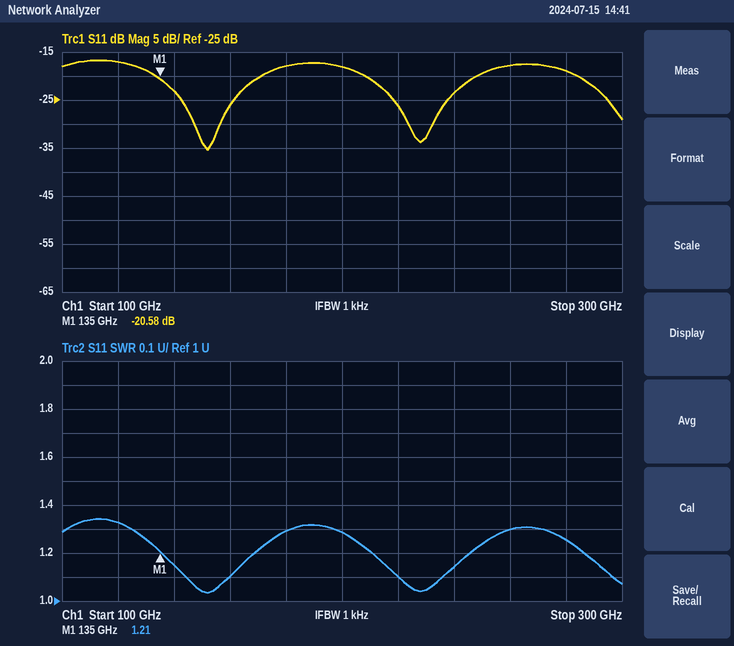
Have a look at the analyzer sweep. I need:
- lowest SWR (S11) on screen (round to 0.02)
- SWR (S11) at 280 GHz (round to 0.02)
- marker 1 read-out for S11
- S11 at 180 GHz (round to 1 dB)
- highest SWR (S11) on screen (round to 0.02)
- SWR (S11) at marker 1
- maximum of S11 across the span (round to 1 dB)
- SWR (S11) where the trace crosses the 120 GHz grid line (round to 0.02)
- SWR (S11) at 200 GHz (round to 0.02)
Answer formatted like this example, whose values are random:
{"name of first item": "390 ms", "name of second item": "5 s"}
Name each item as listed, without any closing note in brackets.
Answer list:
{"lowest SWR (S11) on screen": "1.04", "SWR (S11) at 280 GHz": "1.26", "marker 1 read-out for S11": "-20.58 dB", "S11 at 180 GHz": "-18 dB", "highest SWR (S11) on screen": "1.34", "SWR (S11) at marker 1": "1.21", "maximum of S11 across the span": "-17 dB", "SWR (S11) where the trace crosses the 120 GHz grid line": "1.32", "SWR (S11) at 200 GHz": "1.28"}
